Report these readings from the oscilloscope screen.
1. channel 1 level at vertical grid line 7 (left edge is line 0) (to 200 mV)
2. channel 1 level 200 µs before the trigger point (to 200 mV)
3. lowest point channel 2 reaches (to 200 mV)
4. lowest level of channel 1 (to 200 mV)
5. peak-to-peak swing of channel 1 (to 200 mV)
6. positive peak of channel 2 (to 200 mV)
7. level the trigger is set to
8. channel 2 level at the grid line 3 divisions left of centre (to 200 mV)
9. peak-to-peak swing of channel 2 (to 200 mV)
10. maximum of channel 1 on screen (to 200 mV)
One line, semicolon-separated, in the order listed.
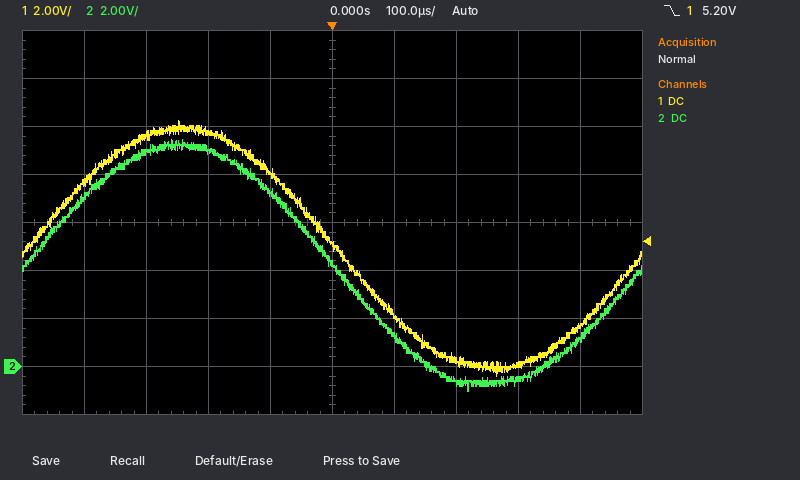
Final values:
200 mV; 9.8 V; -1.0 V; -400 mV; 10.6 V; 9.4 V; 5.20 V; 9.0 V; 10.4 V; 10.2 V
